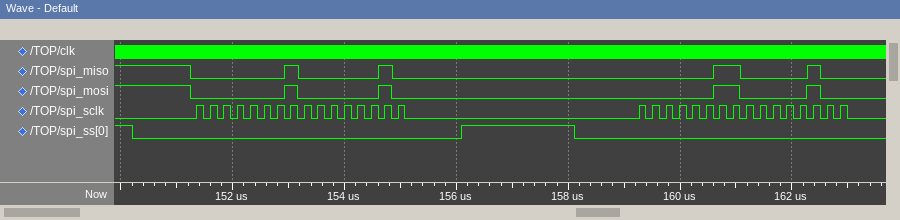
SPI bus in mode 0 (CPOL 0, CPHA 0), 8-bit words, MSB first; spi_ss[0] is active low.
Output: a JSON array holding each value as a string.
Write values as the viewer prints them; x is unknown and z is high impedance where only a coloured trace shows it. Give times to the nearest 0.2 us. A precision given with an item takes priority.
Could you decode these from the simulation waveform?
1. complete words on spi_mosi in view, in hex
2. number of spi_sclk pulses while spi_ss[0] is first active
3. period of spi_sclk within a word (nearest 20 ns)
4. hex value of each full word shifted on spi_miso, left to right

["01, 02, 03, 04", "16", "240 ns", "01, 02, 03, 04"]
